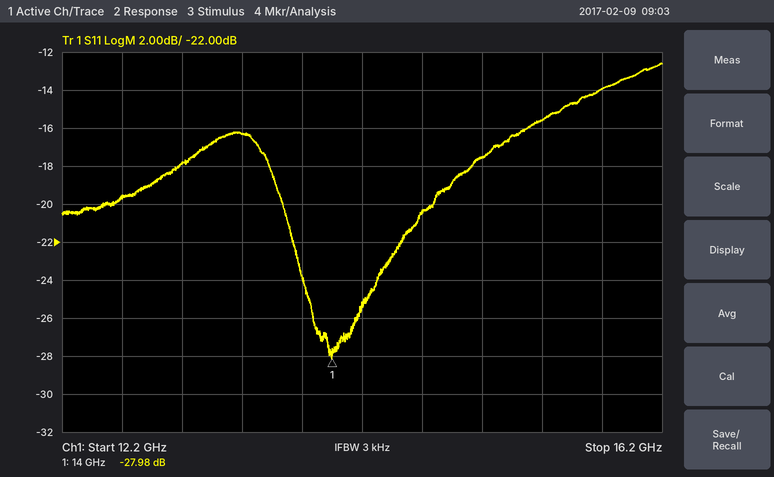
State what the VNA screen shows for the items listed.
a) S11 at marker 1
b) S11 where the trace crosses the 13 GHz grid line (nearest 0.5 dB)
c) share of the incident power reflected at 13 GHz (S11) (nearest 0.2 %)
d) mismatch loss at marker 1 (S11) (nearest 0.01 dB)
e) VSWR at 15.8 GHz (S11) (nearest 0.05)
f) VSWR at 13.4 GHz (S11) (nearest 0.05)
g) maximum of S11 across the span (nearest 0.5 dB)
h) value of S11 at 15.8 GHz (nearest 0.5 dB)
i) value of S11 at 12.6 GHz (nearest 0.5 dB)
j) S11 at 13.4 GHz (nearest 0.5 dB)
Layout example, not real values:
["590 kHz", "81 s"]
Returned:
["-27.98 dB", "-18.0 dB", "1.6 %", "0.01 dB", "1.50", "1.35", "-12.5 dB", "-14.0 dB", "-19.5 dB", "-16.5 dB"]
